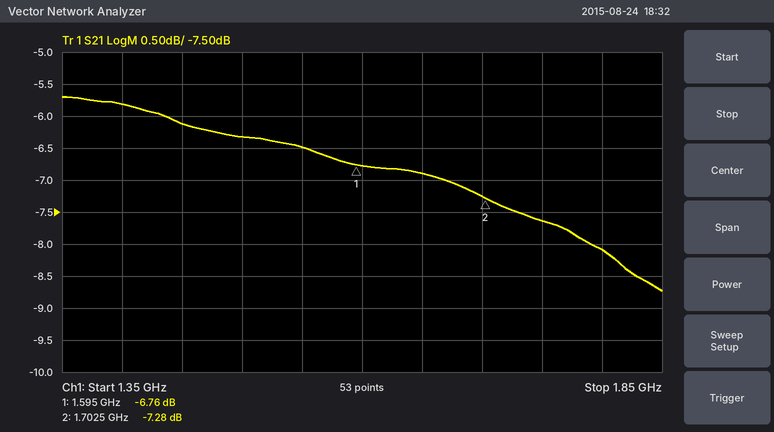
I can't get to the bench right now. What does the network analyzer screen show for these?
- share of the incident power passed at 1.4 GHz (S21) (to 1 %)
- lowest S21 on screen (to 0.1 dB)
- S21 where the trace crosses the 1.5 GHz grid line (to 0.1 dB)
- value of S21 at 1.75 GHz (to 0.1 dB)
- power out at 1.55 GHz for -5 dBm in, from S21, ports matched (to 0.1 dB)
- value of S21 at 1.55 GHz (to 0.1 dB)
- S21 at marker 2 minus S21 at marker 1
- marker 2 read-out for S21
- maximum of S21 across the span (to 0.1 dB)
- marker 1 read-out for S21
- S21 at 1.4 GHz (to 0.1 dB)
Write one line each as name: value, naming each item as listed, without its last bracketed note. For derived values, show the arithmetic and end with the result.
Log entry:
share of the incident power passed at 1.4 GHz (S21): 10^(-5.8/10) ≈ 26 %
lowest S21 on screen: -8.7 dB
S21 where the trace crosses the 1.5 GHz grid line: -6.3 dB
value of S21 at 1.75 GHz: -7.6 dB
power out at 1.55 GHz for -5 dBm in, from S21, ports matched: -5 dBm + (-6.5 dB) = -11.5 dBm
value of S21 at 1.55 GHz: -6.5 dB
S21 at marker 2 minus S21 at marker 1: -7.28 − (-6.76) = -0.52 dB
marker 2 read-out for S21: -7.28 dB
maximum of S21 across the span: -5.7 dB
marker 1 read-out for S21: -6.76 dB
S21 at 1.4 GHz: -5.8 dB
